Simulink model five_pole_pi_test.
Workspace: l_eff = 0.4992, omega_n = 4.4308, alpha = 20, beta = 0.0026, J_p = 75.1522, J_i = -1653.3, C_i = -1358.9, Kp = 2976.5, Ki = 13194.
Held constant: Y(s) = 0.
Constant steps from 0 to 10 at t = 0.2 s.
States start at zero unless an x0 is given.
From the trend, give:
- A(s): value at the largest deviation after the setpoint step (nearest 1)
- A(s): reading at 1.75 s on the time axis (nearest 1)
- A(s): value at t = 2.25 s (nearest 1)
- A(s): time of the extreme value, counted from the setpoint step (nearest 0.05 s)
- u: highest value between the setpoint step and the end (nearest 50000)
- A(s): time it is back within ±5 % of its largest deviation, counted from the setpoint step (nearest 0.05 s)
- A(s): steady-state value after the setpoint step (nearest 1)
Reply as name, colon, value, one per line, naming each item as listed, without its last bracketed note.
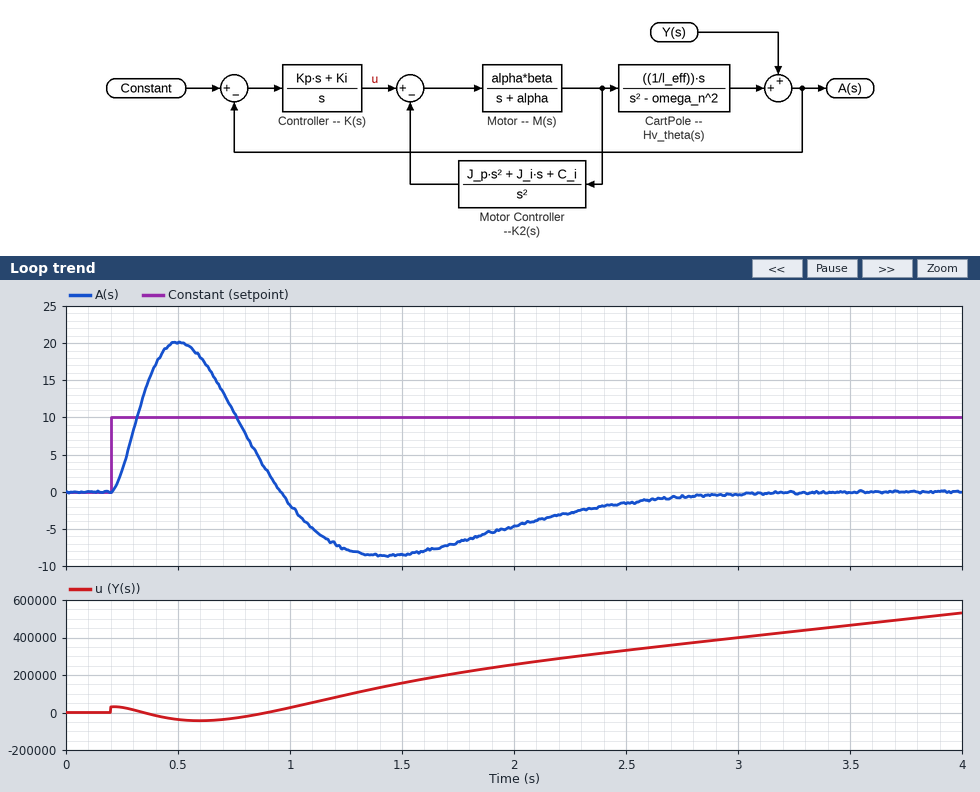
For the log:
A(s): value at the largest deviation after the setpoint step: 20
A(s): reading at 1.75 s on the time axis: -7
A(s): value at t = 2.25 s: -3
A(s): time of the extreme value, counted from the setpoint step: 0.30 s
u: highest value between the setpoint step and the end: 550000
A(s): time it is back within ±5 % of its largest deviation, counted from the setpoint step: 2.45 s
A(s): steady-state value after the setpoint step: 0
